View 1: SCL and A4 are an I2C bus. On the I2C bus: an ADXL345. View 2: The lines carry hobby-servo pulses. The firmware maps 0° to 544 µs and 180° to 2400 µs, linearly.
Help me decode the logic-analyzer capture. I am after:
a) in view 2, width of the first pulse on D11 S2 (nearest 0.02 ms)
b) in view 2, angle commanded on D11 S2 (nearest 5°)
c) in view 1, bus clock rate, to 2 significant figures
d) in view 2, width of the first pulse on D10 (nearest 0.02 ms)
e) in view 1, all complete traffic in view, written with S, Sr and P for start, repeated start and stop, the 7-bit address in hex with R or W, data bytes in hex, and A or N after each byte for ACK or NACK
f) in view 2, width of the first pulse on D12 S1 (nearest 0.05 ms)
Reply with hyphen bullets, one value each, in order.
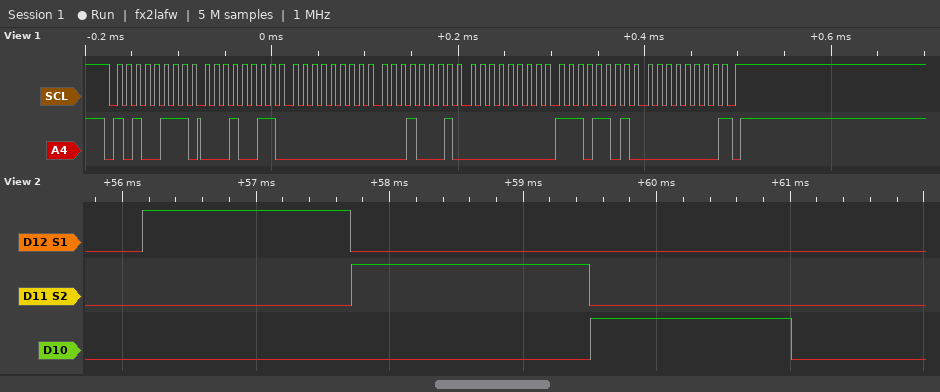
- 1.78 ms
- 120°
- 100 kHz
- 1.50 ms
- S 53R A 13 A 00 A 11 A 00 A ED A 00 N P
- 1.55 ms
